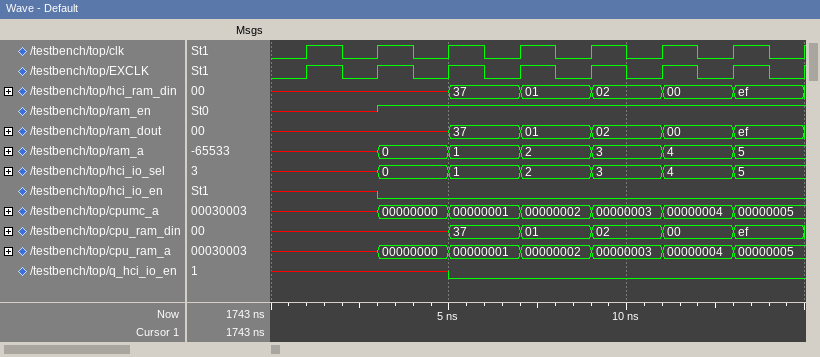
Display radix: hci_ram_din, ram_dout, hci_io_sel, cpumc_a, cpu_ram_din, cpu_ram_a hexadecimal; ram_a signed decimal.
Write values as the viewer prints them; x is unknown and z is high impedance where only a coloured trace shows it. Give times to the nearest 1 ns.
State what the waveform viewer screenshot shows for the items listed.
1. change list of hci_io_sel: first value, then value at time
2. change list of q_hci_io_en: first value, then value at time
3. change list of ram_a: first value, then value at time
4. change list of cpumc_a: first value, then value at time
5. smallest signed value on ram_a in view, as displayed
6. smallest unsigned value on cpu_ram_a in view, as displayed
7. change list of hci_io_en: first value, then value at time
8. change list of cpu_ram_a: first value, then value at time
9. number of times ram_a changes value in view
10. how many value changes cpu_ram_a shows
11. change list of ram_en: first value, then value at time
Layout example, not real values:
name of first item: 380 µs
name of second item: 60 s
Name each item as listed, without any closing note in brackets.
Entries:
change list of hci_io_sel: first value, then value at time: x, 0 at 3 ns, 1 at 5 ns, 2 at 7 ns, 3 at 9 ns, 4 at 11 ns, 5 at 13 ns
change list of q_hci_io_en: first value, then value at time: x, 0 at 5 ns
change list of ram_a: first value, then value at time: x, 0 at 3 ns, 1 at 5 ns, 2 at 7 ns, 3 at 9 ns, 4 at 11 ns, 5 at 13 ns
change list of cpumc_a: first value, then value at time: x, 00000000 at 3 ns, 00000001 at 5 ns, 00000002 at 7 ns, 00000003 at 9 ns, 00000004 at 11 ns, 00000005 at 13 ns
smallest signed value on ram_a in view, as displayed: 0
smallest unsigned value on cpu_ram_a in view, as displayed: 00000000
change list of hci_io_en: first value, then value at time: x, 0 at 3 ns
change list of cpu_ram_a: first value, then value at time: x, 00000000 at 3 ns, 00000001 at 5 ns, 00000002 at 7 ns, 00000003 at 9 ns, 00000004 at 11 ns, 00000005 at 13 ns
number of times ram_a changes value in view: 6
how many value changes cpu_ram_a shows: 6
change list of ram_en: first value, then value at time: x, 1 at 3 ns
